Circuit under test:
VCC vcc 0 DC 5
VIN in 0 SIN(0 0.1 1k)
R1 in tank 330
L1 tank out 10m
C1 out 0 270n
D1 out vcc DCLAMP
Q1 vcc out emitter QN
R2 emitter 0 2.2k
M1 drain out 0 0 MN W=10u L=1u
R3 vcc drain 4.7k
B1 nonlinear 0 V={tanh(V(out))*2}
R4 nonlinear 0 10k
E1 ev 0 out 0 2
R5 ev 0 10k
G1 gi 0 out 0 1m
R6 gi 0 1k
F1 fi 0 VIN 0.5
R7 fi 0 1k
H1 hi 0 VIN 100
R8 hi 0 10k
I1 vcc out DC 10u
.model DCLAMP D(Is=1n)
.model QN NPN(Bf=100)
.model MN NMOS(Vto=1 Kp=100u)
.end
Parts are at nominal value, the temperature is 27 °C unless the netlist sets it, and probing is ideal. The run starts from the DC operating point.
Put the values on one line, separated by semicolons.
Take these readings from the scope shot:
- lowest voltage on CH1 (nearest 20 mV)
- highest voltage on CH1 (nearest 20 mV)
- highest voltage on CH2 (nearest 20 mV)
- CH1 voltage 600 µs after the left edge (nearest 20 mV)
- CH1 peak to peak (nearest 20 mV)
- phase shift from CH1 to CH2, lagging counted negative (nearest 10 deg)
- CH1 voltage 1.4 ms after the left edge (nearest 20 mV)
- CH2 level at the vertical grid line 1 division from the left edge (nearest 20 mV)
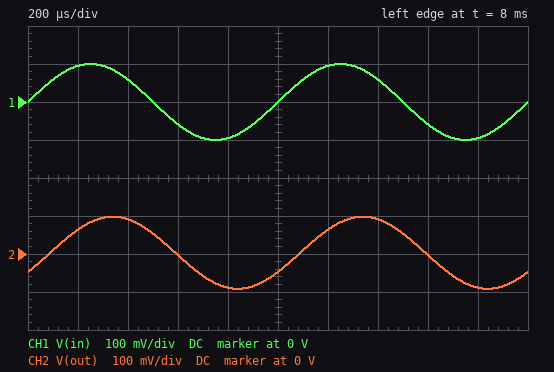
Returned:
-100 mV; 100 mV; 100 mV; -60 mV; 200 mV; -30 deg; 60 mV; 60 mV
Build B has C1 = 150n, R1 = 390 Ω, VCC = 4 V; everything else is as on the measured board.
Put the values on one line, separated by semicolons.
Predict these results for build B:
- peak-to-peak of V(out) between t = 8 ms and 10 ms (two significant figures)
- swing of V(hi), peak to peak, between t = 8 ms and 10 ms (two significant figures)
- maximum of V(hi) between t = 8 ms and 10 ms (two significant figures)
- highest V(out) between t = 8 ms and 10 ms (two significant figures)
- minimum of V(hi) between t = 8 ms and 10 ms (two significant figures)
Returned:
200 mV; 19 mV; 10 mV; 100 mV; -8.3 mV
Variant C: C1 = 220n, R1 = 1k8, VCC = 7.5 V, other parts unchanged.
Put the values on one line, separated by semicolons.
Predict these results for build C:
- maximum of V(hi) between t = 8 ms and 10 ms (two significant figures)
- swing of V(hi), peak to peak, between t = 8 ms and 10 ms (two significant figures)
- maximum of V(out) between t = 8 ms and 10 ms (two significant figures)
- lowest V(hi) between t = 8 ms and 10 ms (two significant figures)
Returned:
6.2 mV; 10 mV; 56 mV; -4.2 mV
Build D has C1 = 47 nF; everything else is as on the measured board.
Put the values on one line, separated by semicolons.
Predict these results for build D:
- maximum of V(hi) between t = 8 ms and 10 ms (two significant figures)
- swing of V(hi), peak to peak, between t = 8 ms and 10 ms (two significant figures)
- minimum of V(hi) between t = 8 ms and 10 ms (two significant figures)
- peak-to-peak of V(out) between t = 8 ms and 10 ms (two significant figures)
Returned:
4.0 mV; 6.0 mV; -2.0 mV; 200 mV
